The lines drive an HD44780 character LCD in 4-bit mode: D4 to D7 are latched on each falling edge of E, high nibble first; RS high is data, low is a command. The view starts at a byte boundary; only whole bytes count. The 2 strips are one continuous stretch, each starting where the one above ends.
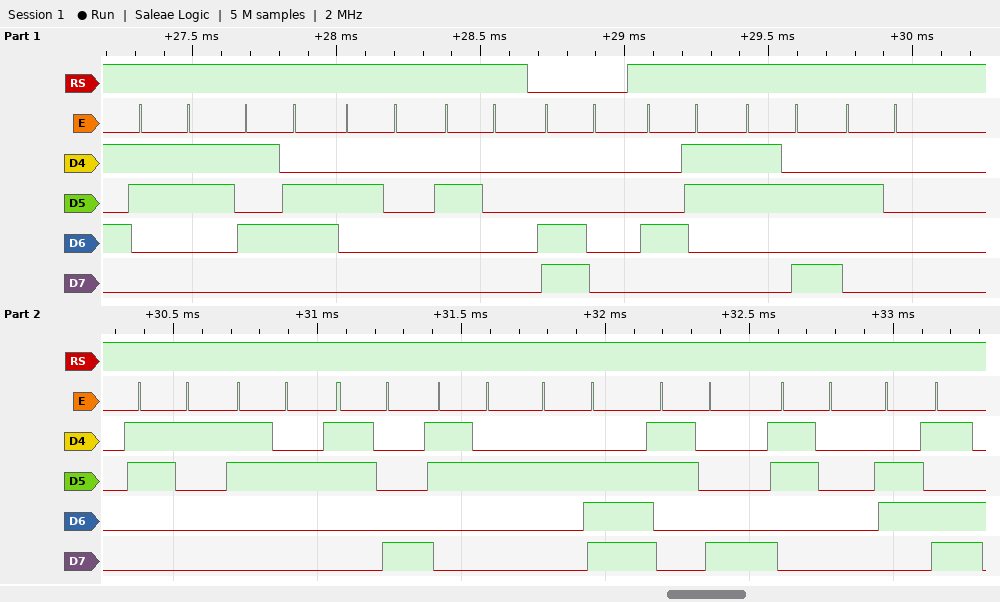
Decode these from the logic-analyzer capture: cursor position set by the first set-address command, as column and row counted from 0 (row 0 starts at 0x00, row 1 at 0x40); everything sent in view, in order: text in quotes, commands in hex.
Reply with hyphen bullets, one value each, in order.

- column 0, row 1
- "3V  " 0xC0 "C: 1282.80m"
